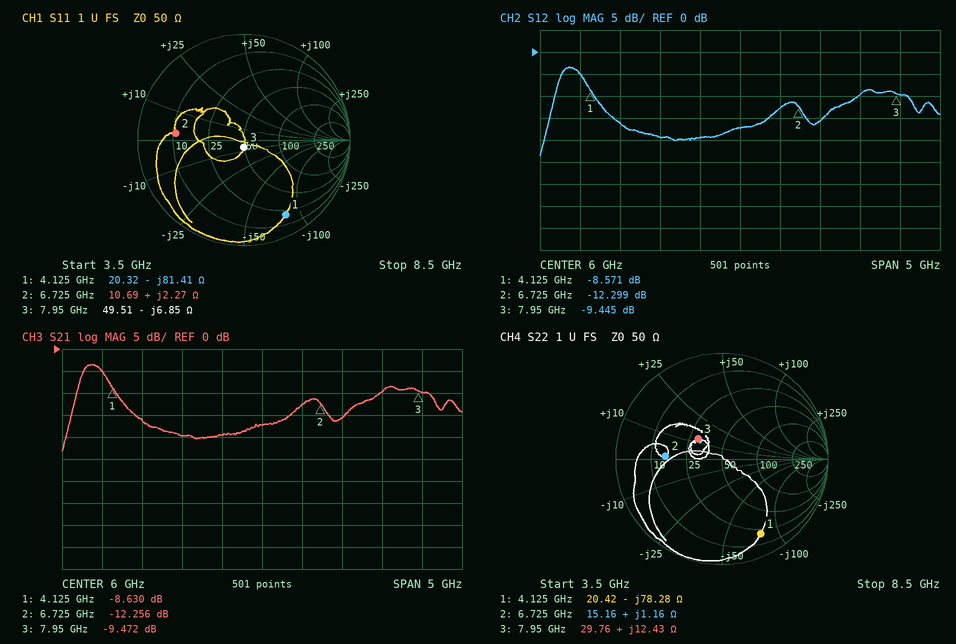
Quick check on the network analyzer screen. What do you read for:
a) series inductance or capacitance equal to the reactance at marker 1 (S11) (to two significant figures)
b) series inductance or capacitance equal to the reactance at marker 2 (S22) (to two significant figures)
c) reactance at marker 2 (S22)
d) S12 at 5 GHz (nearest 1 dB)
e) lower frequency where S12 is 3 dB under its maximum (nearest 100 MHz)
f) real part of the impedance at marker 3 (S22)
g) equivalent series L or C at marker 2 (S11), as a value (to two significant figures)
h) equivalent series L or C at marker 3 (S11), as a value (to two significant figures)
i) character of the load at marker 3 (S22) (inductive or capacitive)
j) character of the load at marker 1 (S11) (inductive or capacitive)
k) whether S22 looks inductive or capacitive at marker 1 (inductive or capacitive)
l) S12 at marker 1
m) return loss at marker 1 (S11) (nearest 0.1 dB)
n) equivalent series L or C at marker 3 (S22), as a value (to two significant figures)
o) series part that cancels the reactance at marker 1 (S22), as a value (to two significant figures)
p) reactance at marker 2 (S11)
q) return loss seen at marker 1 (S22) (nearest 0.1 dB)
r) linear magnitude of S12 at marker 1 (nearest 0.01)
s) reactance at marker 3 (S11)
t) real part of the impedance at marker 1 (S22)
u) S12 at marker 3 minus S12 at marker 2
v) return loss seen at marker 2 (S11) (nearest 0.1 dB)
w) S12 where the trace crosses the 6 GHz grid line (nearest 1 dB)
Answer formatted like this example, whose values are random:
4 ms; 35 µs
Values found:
470 fF; 27 pH; +1.16 Ω; -19 dB; 3.7 GHz; 29.76 Ω; 54 pH; 2.9 pF; inductive; capacitive; capacitive; -8.571 dB; 1.9 dB; 250 pH; 3.0 nH; +2.27 Ω; 2.0 dB; 0.37; -6.85 Ω; 20.42 Ω; 2.854 dB; 3.8 dB; -17 dB
